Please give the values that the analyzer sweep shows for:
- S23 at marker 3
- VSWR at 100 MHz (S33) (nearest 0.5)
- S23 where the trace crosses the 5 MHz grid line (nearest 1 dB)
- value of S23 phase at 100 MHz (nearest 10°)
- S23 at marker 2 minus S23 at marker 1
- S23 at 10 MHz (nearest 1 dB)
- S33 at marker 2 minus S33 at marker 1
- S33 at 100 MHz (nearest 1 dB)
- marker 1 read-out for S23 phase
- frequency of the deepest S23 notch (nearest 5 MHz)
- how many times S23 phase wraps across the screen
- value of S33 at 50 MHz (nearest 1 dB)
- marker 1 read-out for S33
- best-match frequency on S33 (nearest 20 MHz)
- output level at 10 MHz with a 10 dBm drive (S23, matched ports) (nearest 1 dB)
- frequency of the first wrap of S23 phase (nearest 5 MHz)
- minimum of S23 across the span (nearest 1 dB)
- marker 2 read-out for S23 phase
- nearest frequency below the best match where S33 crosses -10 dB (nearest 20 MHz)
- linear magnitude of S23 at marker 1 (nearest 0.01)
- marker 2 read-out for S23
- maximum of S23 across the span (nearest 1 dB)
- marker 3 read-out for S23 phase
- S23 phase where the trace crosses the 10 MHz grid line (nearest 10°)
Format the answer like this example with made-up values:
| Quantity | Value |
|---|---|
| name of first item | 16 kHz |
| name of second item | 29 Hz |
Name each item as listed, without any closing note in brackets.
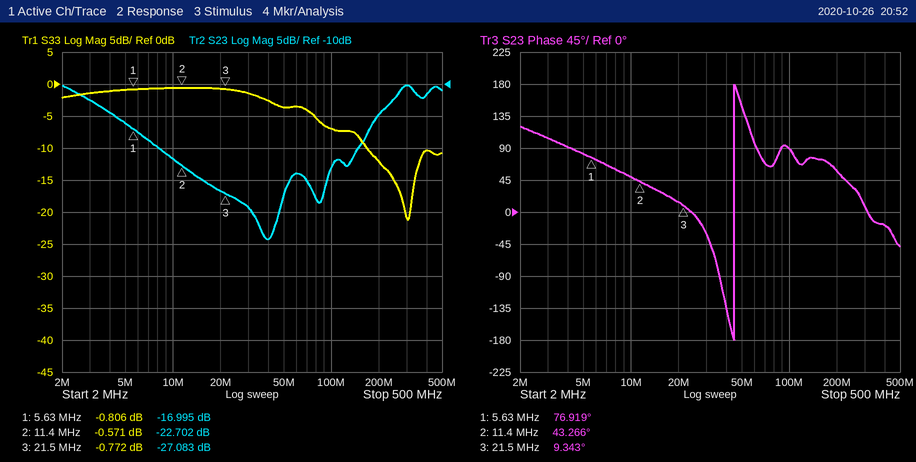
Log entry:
| Quantity | Value |
|---|---|
| S23 at marker 3 | -27.083 dB |
| VSWR at 100 MHz (S33) | 2.5 |
| S23 where the trace crosses the 5 MHz grid line | -16 dB |
| value of S23 phase at 100 MHz | 90° |
| S23 at marker 2 minus S23 at marker 1 | -5.707 dB |
| S23 at 10 MHz | -22 dB |
| S33 at marker 2 minus S33 at marker 1 | 0.235 dB |
| S33 at 100 MHz | -7 dB |
| marker 1 read-out for S23 phase | 76.919° |
| frequency of the deepest S23 notch | 40 MHz |
| how many times S23 phase wraps across the screen | 1 |
| value of S33 at 50 MHz | -4 dB |
| marker 1 read-out for S33 | -0.806 dB |
| best-match frequency on S33 | 300 MHz |
| output level at 10 MHz with a 10 dBm drive (S23, matched ports) | -12 dBm |
| frequency of the first wrap of S23 phase | 45 MHz |
| minimum of S23 across the span | -34 dB |
| marker 2 read-out for S23 phase | 43.266° |
| nearest frequency below the best match where S33 crosses -10 dB | 160 MHz |
| linear magnitude of S23 at marker 1 | 0.14 |
| marker 2 read-out for S23 | -22.702 dB |
| maximum of S23 across the span | -10 dB |
| marker 3 read-out for S23 phase | 9.343° |
| S23 phase where the trace crosses the 10 MHz grid line | 50° |
